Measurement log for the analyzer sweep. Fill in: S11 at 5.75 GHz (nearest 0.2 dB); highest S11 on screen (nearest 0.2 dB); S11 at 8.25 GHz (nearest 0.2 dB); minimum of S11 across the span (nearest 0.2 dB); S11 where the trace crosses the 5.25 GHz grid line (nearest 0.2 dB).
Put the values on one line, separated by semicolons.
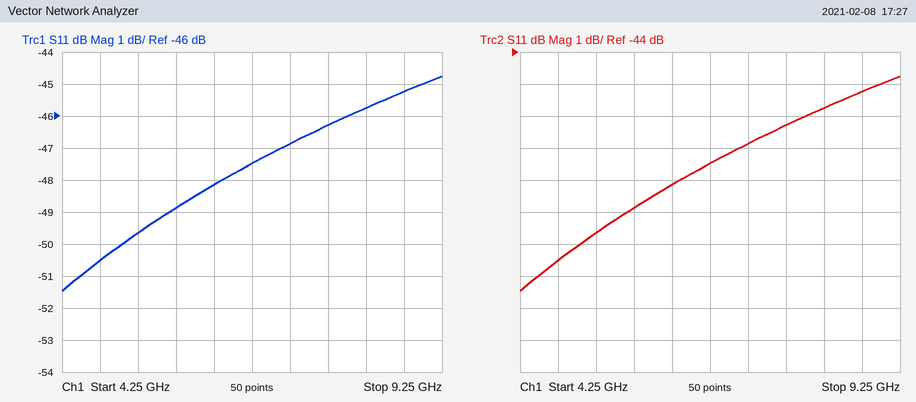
-48.8 dB; -44.8 dB; -45.8 dB; -51.4 dB; -49.6 dB
